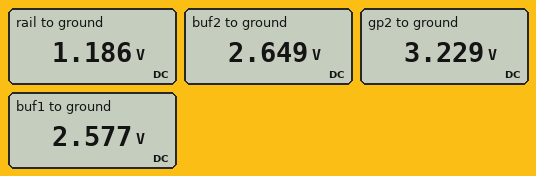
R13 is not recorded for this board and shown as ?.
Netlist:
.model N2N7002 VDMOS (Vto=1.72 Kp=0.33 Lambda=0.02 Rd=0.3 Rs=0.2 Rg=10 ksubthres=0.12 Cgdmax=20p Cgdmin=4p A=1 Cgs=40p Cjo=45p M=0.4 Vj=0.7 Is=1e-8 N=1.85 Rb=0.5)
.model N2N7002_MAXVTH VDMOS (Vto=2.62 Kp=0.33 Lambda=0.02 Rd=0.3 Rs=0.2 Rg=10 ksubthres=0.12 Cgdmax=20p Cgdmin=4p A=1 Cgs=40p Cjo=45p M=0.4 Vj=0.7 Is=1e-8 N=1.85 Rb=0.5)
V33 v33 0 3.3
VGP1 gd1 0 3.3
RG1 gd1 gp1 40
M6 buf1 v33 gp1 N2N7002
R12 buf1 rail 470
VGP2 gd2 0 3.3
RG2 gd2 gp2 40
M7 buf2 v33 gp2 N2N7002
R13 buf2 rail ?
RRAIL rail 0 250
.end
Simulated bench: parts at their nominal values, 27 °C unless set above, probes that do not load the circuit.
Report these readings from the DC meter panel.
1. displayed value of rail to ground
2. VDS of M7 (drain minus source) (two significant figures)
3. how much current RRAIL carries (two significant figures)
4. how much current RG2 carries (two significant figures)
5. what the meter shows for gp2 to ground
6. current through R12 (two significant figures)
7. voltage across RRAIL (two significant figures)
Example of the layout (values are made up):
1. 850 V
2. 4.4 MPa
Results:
1. 1.186 V
2. -580 mV
3. 4.7 mA
4. 1.8 mA
5. 3.229 V
6. 3.0 mA
7. 1.2 V
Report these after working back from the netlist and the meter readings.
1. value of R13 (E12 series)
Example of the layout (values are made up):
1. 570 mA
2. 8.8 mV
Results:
1. 820 Ω
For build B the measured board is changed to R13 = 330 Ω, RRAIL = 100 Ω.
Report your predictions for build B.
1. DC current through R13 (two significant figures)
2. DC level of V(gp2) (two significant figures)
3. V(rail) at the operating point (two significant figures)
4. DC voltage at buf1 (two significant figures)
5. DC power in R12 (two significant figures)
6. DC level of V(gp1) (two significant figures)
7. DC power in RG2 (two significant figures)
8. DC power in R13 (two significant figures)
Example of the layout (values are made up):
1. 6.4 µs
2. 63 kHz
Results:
1. 4.9 mA
2. 3.1 V
3. 850 mV
4. 2.5 V
5. 6.1 mW
6. 3.2 V
7. 970 µW
8. 8.0 mW
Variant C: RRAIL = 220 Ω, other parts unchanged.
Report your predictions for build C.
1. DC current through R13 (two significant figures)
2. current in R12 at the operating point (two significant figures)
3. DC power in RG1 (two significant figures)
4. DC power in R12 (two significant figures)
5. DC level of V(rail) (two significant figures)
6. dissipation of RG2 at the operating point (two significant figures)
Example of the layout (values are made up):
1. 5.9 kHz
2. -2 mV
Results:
1. 1.9 mA
2. 3.1 mA
3. 390 µW
4. 4.6 mW
5. 1.1 V
6. 140 µW
